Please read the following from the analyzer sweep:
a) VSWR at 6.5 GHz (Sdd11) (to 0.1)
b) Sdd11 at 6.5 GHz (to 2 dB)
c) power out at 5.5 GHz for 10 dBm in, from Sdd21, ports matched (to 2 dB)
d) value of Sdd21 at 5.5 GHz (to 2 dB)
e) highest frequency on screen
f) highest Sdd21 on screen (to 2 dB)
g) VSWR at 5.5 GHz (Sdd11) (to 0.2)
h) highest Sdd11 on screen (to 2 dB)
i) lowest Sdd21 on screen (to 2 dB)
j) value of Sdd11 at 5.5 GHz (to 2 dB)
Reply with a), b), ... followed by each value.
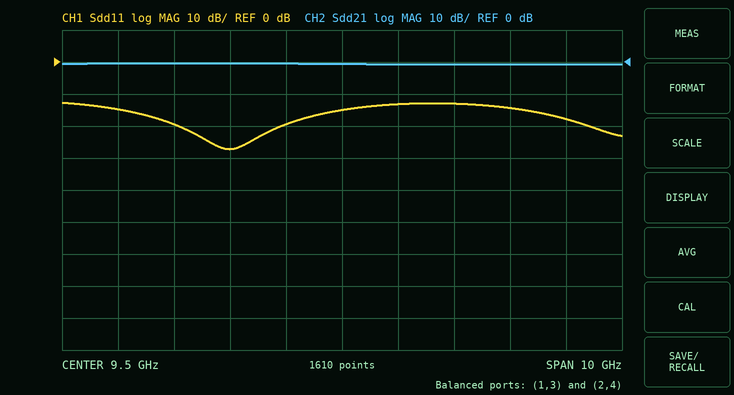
a) 1.2
b) -20 dB
c) 10 dBm
d) 0 dB
e) 14.5 GHz
f) 0 dB
g) 1.4
h) -12 dB
i) 0 dB
j) -14 dB
